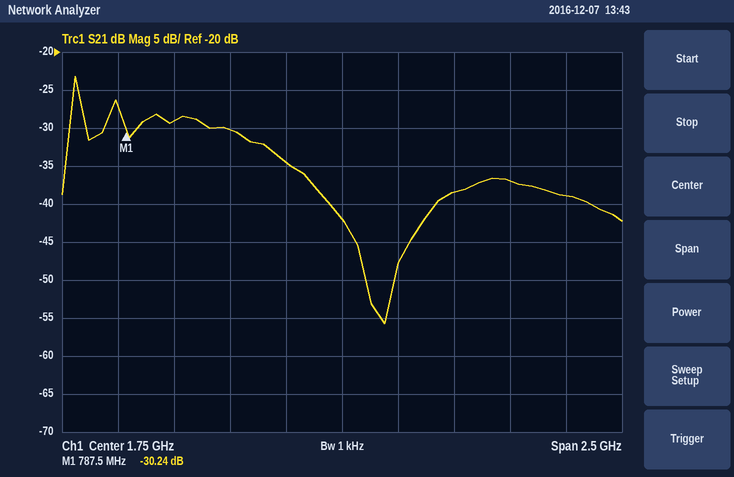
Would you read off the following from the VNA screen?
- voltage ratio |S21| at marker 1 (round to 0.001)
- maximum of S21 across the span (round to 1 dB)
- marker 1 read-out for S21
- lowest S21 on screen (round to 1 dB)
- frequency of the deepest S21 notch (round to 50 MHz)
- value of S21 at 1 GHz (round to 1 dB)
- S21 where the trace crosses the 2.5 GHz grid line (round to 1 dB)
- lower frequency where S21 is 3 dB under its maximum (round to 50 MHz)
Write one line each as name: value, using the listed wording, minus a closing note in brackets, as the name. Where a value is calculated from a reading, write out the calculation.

voltage ratio |S21| at marker 1: 10^(-30.24/20) ≈ 0.031
maximum of S21 across the span: -23 dB
marker 1 read-out for S21: -30.24 dB
lowest S21 on screen: -56 dB
frequency of the deepest S21 notch: 1.95 GHz
value of S21 at 1 GHz: -29 dB
S21 where the trace crosses the 2.5 GHz grid line: -37 dB
lower frequency where S21 is 3 dB under its maximum: 550 MHz
